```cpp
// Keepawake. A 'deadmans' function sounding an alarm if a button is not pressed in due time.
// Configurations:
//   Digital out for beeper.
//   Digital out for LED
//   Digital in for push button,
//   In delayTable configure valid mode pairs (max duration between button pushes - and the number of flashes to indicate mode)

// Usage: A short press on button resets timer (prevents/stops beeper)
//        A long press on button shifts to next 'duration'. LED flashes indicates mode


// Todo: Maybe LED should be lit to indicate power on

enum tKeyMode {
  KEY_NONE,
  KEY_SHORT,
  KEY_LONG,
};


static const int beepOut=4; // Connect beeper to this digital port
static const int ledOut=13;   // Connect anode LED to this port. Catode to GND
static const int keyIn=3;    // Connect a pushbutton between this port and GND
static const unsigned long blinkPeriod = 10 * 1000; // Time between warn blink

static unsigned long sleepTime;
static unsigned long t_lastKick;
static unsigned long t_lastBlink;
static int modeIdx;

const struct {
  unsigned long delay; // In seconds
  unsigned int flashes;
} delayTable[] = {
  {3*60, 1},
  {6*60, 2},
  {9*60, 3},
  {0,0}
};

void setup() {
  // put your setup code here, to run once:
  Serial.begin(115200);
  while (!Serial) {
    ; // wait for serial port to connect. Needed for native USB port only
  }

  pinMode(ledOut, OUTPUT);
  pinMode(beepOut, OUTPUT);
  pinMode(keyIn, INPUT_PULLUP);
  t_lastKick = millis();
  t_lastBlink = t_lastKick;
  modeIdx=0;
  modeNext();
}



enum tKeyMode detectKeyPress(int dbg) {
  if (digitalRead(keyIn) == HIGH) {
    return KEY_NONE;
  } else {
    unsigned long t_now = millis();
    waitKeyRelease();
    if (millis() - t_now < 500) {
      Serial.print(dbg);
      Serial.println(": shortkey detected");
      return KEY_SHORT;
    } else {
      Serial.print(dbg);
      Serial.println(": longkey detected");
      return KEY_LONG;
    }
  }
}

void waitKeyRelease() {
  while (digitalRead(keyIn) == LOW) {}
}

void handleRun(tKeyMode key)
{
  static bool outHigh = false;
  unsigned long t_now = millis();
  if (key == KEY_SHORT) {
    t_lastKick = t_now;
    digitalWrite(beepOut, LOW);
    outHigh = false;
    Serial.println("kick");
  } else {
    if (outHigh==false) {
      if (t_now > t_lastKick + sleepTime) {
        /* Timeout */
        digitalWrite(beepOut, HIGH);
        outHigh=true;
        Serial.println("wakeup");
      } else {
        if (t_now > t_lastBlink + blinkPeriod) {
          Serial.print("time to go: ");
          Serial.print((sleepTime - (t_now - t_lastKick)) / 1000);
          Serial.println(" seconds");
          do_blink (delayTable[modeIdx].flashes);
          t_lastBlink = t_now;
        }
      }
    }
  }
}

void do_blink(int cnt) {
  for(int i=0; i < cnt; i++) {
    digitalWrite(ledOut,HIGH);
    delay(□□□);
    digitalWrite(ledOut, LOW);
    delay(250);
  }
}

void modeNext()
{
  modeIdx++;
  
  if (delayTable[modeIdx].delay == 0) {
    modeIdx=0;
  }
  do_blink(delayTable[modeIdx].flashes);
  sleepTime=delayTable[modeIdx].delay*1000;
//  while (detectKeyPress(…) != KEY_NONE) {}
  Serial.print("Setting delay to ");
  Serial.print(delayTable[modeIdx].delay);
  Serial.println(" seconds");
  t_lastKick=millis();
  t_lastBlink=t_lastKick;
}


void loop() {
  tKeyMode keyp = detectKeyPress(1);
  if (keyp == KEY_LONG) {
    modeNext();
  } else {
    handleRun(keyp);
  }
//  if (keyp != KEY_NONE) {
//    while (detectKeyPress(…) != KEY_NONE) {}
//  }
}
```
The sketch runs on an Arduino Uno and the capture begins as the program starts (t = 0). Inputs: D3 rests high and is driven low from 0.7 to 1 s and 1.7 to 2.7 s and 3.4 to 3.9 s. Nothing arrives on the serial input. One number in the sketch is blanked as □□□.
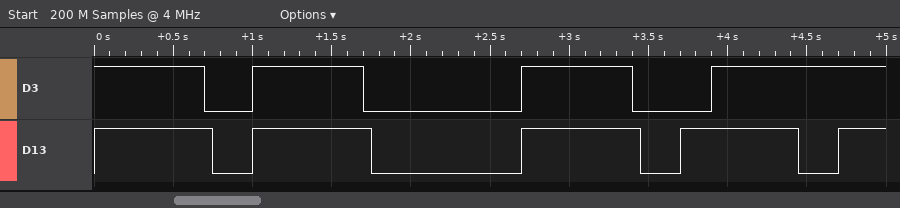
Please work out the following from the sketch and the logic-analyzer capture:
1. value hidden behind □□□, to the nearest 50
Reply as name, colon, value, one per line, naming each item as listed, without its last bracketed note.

value hidden behind □□□, to the nearest 50: 750
